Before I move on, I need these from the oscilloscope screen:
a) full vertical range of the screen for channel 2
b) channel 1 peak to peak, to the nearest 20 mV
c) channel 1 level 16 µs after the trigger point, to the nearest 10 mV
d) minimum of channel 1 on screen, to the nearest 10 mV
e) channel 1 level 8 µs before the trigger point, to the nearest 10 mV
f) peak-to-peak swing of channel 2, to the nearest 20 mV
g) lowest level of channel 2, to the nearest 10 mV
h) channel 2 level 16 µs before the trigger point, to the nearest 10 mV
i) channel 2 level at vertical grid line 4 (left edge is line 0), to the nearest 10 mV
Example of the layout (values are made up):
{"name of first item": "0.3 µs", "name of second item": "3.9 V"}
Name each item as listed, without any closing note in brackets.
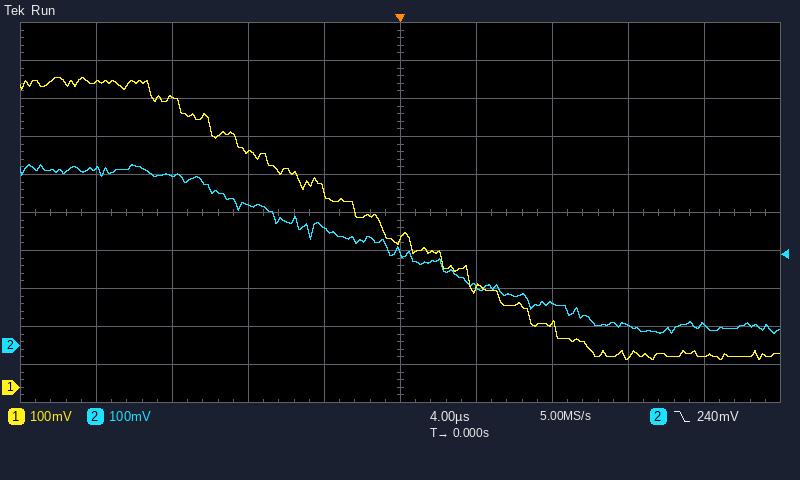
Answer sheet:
{"full vertical range of the screen for channel 2": "1 V", "channel 1 peak to peak, to the nearest 20 mV": "740 mV", "channel 1 level 16 µs after the trigger point, to the nearest 10 mV": "80 mV", "minimum of channel 1 on screen, to the nearest 10 mV": "70 mV", "channel 1 level 8 µs before the trigger point, to the nearest 10 mV": "620 mV", "peak-to-peak swing of channel 2, to the nearest 20 mV": "440 mV", "lowest level of channel 2, to the nearest 10 mV": "30 mV", "channel 2 level 16 µs before the trigger point, to the nearest 10 mV": "460 mV", "channel 2 level at vertical grid line 4 (left edge is line 0), to the nearest 10 mV": "310 mV"}
